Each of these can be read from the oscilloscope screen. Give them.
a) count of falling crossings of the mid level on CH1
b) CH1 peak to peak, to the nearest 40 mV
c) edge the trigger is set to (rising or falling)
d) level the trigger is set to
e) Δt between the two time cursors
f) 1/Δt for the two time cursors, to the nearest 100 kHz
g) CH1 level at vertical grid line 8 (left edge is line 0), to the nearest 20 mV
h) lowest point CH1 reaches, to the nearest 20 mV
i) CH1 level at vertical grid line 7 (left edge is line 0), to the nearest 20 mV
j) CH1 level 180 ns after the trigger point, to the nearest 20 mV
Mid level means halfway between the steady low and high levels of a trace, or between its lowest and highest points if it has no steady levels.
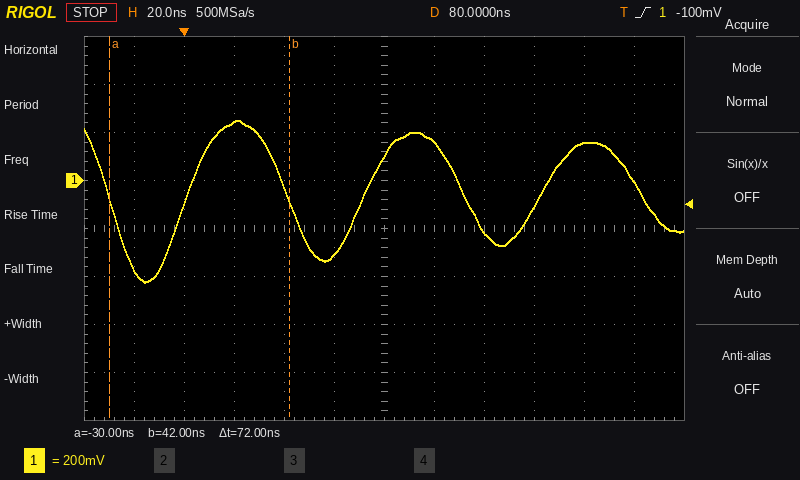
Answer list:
4
680 mV
rising
-100 mV
72 ns
13.9 MHz
-220 mV
-420 mV
160 mV
0 mV
